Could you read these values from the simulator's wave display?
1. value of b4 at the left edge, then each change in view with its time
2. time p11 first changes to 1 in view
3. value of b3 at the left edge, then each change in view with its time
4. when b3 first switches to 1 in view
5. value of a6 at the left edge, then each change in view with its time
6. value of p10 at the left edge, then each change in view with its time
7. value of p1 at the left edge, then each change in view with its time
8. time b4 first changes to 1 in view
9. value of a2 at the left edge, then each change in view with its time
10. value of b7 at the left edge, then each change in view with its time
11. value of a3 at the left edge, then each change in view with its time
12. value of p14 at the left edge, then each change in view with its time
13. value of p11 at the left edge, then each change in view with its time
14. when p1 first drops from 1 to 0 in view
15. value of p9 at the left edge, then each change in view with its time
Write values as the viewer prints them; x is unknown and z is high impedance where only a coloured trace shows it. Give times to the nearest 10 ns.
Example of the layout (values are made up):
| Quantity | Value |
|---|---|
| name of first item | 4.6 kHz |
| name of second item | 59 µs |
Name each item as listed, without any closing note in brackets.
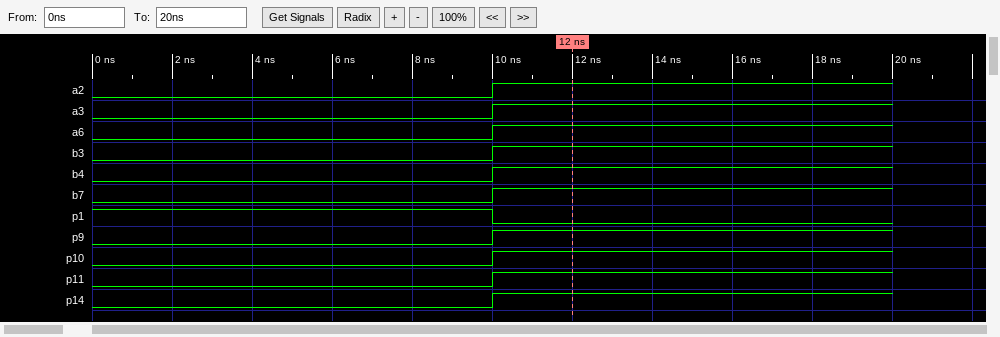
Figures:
| Quantity | Value |
|---|---|
| value of b4 at the left edge, then each change in view with its time | 0, 1 at 10 ns |
| time p11 first changes to 1 in view | 10 ns |
| value of b3 at the left edge, then each change in view with its time | 0, 1 at 10 ns |
| when b3 first switches to 1 in view | 10 ns |
| value of a6 at the left edge, then each change in view with its time | 0, 1 at 10 ns |
| value of p10 at the left edge, then each change in view with its time | 0, 1 at 10 ns |
| value of p1 at the left edge, then each change in view with its time | 1, 0 at 10 ns |
| time b4 first changes to 1 in view | 10 ns |
| value of a2 at the left edge, then each change in view with its time | 0, 1 at 10 ns |
| value of b7 at the left edge, then each change in view with its time | 0, 1 at 10 ns |
| value of a3 at the left edge, then each change in view with its time | 0, 1 at 10 ns |
| value of p14 at the left edge, then each change in view with its time | 0, 1 at 10 ns |
| value of p11 at the left edge, then each change in view with its time | 0, 1 at 10 ns |
| when p1 first drops from 1 to 0 in view | 10 ns |
| value of p9 at the left edge, then each change in view with its time | 0, 1 at 10 ns |
